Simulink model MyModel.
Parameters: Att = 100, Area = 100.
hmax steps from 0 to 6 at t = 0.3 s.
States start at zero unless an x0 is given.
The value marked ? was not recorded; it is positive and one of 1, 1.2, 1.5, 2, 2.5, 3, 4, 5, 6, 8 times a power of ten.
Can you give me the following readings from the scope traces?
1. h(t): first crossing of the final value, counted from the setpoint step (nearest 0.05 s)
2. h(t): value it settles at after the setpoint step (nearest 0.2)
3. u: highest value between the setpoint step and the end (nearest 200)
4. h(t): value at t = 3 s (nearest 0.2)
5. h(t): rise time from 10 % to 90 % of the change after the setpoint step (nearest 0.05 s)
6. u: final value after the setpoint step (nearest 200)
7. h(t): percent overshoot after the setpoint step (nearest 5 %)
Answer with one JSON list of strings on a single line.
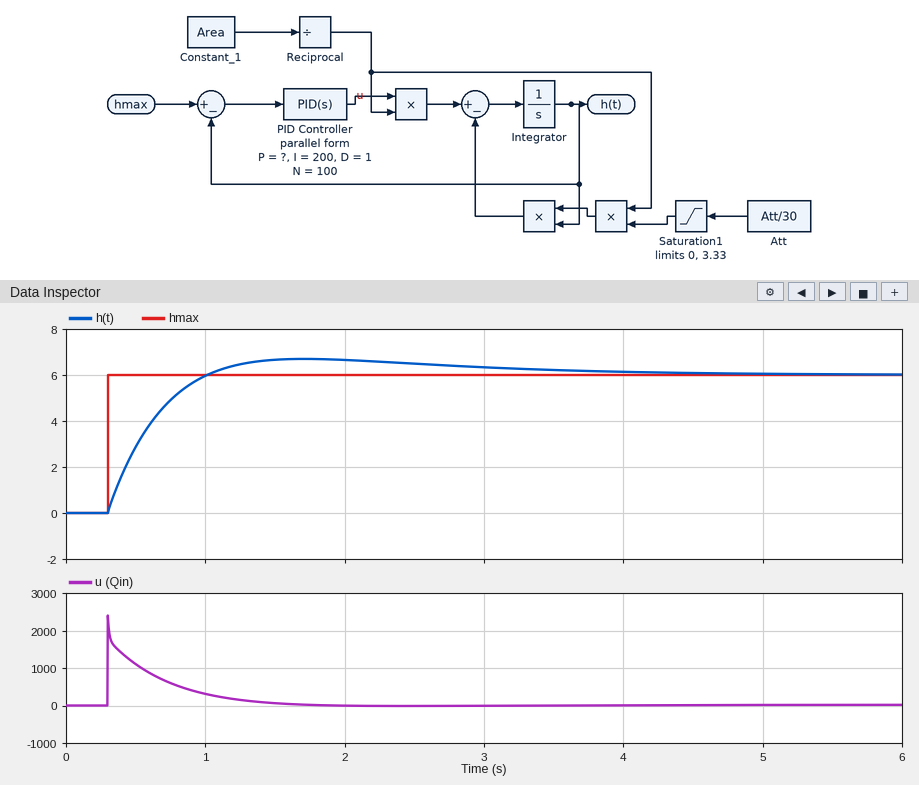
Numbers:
["0.70 s", "6.0", "2400", "6.4", "0.50 s", "0", "10 %"]
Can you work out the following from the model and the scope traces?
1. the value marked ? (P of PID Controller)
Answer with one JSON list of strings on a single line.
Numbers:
["300"]
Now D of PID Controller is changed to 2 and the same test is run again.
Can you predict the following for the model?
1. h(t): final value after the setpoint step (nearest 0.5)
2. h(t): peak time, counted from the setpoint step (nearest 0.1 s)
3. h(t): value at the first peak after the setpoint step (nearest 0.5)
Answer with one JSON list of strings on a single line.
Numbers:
["6.0", "1.4 s", "6.5"]
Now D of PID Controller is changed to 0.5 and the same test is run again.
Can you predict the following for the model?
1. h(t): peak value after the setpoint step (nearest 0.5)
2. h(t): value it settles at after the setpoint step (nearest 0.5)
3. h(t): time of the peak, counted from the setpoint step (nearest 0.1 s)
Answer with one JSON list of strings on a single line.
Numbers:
["6.5", "6.0", "1.4 s"]
